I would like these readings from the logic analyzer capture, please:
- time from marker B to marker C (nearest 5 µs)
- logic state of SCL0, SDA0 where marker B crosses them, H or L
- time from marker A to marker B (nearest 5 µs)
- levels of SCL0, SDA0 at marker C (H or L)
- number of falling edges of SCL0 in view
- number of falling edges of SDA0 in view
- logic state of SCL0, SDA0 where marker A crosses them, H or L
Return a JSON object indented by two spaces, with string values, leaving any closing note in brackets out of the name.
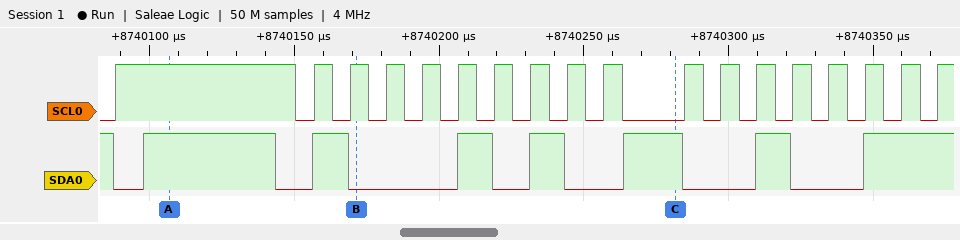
{
  "time from marker B to marker C": "110 µs",
  "logic state of SCL0, SDA0 where marker B crosses them, H or L": "SCL0=H, SDA0=L",
  "time from marker A to marker B": "65 µs",
  "levels of SCL0, SDA0 at marker C": "SCL0=L, SDA0=H",
  "number of falling edges of SCL0 in view": "17",
  "number of falling edges of SDA0 in view": "7",
  "logic state of SCL0, SDA0 where marker A crosses them, H or L": "SCL0=H, SDA0=H"
}
